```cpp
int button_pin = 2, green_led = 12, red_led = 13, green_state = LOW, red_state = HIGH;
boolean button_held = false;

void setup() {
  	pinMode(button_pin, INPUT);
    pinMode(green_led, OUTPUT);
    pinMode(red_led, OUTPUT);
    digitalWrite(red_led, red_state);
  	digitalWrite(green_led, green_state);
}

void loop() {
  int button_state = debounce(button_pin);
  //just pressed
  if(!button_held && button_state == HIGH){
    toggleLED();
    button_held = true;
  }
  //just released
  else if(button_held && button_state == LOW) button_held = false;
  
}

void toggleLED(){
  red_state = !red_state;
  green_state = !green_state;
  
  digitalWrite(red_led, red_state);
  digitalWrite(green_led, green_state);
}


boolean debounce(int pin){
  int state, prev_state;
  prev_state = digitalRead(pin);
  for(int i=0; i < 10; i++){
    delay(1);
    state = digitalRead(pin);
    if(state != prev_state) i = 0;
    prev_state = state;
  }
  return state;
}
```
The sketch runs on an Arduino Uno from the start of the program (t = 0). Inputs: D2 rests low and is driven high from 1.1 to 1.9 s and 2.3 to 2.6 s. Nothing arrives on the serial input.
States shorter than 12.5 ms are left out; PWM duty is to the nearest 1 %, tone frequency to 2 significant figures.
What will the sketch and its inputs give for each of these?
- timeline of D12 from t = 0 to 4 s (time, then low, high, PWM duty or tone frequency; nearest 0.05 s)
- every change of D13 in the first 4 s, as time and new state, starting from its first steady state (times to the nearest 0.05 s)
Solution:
0 s low; 1.1 s high; 2.3 s low
0 s high; 1.1 s low; 2.3 s high
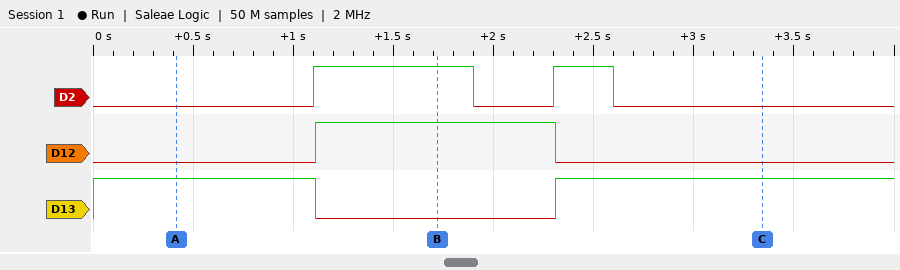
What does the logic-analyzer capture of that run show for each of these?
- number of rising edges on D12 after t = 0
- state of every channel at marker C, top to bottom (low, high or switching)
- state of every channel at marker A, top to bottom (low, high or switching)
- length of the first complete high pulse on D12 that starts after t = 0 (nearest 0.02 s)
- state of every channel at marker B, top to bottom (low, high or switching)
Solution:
1
D2 low, D12 low, D13 high
D2 low, D12 low, D13 high
1.20 s
D2 high, D12 high, D13 low
